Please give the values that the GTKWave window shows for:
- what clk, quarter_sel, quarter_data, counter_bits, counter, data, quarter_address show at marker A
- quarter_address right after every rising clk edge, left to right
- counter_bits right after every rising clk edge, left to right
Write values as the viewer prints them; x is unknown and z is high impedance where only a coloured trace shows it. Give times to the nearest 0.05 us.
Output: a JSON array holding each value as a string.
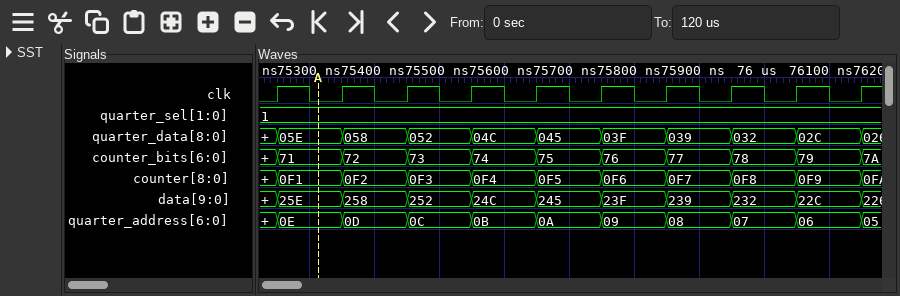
["clk=0, quarter_sel=1, quarter_data=05E, counter_bits=71, counter=0F1, data=25E, quarter_address=0E", "0E, 0D, 0C, 0B, 0A, 09, 08, 07, 06, 05", "71, 72, 73, 74, 75, 76, 77, 78, 79, 7A"]
